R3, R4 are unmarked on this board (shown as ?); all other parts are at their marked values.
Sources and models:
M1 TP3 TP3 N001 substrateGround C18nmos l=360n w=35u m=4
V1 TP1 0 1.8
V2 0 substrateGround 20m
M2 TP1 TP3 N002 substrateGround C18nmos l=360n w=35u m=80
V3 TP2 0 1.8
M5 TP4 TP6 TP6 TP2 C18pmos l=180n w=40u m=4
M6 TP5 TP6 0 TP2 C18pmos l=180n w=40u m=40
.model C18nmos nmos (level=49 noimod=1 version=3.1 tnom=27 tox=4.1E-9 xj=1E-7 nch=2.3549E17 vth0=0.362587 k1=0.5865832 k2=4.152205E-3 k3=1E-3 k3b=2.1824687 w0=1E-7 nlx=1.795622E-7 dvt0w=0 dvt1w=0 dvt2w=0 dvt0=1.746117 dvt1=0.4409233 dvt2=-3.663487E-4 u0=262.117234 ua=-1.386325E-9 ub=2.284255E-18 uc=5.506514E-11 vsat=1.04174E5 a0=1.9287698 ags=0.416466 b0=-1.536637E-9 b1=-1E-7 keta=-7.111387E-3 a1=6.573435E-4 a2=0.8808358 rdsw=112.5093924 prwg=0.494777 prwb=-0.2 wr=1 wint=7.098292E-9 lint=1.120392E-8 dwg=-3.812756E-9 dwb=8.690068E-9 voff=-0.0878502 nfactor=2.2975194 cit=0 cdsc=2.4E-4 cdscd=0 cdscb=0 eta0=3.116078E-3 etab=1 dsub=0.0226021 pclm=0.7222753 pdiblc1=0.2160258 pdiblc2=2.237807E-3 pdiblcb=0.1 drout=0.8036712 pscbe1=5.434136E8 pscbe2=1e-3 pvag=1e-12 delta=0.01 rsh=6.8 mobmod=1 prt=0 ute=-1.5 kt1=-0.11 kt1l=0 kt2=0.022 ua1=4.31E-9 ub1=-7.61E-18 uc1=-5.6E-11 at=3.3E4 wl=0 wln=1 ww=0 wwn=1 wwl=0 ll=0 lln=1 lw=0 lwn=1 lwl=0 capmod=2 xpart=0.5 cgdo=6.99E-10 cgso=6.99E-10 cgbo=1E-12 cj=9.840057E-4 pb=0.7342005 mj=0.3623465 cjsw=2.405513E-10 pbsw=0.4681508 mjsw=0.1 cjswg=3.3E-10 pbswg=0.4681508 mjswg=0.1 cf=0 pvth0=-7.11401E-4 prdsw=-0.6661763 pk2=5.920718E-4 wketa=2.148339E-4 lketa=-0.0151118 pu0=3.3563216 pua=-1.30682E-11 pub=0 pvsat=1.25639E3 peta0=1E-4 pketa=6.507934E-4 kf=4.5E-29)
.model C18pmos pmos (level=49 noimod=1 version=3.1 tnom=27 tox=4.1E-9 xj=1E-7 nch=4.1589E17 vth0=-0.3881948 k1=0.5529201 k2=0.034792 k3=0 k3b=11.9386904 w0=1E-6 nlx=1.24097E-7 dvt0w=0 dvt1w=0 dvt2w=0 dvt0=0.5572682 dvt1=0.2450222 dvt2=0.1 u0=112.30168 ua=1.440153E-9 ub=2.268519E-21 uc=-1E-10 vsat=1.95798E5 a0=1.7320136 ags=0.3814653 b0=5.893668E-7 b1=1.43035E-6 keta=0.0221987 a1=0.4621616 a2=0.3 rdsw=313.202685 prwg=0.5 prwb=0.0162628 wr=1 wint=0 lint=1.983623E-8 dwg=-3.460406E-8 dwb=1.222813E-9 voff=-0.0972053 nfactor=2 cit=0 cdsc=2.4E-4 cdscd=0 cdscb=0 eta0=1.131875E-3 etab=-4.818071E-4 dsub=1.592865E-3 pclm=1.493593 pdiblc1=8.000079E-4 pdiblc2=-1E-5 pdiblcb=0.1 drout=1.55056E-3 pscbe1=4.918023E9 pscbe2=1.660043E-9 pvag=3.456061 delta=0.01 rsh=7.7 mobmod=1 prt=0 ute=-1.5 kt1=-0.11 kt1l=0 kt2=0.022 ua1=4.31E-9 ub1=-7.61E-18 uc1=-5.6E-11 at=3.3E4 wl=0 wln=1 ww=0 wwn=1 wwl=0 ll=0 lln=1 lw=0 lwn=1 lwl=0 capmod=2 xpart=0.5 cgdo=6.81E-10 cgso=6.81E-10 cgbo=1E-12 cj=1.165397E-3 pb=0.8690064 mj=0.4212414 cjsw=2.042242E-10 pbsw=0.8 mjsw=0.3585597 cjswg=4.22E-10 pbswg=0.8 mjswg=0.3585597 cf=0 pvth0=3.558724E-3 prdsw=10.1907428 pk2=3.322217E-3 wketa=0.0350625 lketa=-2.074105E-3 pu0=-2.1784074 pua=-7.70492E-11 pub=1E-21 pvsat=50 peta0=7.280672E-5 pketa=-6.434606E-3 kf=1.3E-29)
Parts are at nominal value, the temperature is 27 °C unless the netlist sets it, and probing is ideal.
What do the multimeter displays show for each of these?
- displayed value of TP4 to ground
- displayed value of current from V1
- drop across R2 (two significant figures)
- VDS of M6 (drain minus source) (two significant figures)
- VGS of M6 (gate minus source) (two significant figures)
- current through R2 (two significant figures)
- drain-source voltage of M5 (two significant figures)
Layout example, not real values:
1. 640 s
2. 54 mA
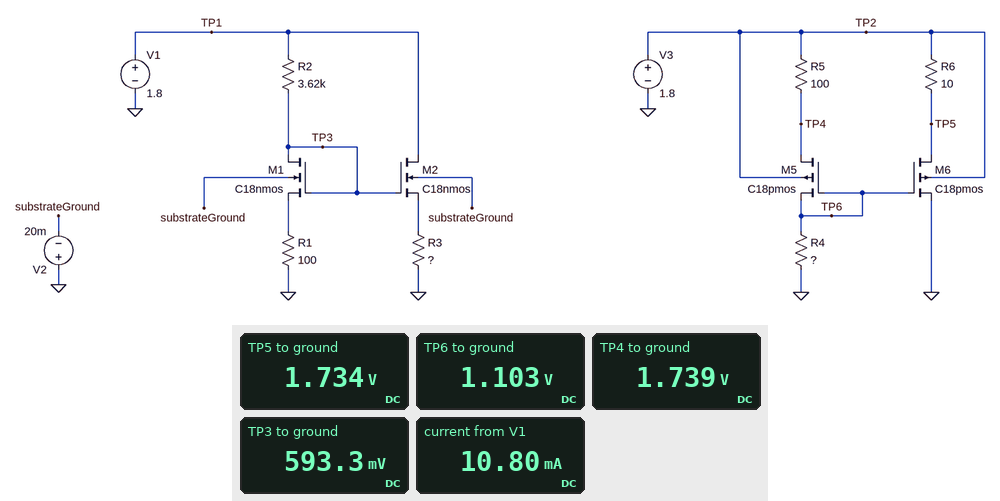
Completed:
1. 1.739 V
2. 10.80 mA
3. 1.2 V
4. 1.7 V
5. 1.1 V
6. 330 µA
7. 640 mV
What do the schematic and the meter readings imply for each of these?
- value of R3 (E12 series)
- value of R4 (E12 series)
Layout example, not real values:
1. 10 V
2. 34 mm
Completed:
1. 1.8 Ω
2. 1.8 kΩ
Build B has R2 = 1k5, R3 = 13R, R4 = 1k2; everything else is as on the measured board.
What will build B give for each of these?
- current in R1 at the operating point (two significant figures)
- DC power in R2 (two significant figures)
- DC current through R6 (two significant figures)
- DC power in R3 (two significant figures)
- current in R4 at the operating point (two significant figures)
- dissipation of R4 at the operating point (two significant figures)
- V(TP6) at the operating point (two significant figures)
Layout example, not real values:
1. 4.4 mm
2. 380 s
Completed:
1. 740 µA
2. 820 µW
3. 9.2 mA
4. 890 µW
5. 870 µA
6. 910 µW
7. 1.0 V
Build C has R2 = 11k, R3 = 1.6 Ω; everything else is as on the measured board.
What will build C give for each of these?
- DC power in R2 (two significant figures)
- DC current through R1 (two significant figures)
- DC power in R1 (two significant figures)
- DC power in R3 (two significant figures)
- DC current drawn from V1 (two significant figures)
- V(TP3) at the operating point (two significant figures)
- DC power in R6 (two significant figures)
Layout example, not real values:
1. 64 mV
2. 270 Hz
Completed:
1. 150 µW
2. 120 µA
3. 1.4 µW
4. 18 µW
5. 3.5 mA
6. 510 mV
7. 430 µW
